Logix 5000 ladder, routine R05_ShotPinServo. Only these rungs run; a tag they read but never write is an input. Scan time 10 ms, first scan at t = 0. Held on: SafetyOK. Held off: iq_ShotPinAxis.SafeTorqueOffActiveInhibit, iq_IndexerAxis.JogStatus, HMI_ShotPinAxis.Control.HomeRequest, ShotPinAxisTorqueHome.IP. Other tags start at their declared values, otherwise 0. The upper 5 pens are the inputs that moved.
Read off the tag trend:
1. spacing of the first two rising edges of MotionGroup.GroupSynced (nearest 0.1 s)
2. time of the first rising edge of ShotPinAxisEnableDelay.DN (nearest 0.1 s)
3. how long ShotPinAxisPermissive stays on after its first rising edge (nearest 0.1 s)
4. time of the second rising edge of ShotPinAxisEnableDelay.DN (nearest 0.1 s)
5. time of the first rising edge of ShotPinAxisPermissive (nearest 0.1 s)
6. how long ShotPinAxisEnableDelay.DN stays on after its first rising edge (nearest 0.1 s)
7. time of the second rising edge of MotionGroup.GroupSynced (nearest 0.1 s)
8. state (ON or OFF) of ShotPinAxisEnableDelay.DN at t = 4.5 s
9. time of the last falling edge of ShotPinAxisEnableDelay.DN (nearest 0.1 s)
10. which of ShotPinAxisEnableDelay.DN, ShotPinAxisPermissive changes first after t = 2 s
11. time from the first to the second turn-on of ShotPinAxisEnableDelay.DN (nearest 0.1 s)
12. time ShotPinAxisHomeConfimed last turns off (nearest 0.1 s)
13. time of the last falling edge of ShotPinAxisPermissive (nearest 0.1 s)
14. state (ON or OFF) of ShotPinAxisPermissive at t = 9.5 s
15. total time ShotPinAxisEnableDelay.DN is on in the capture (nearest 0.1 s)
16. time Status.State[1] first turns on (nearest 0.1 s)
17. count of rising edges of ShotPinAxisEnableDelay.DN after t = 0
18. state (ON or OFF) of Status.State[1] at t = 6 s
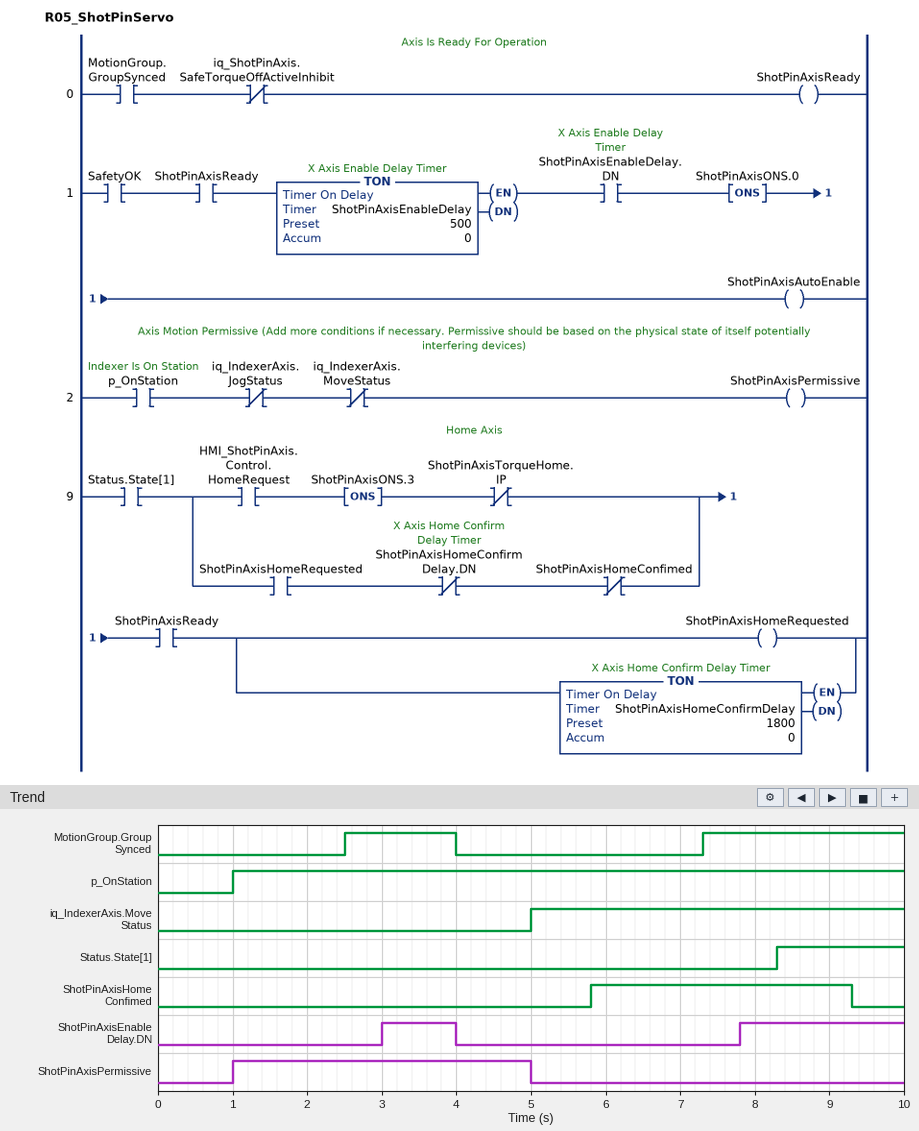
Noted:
4.8 s
3.0 s
4.0 s
7.8 s
1.0 s
1.0 s
7.3 s
OFF
4.0 s
ShotPinAxisEnableDelay.DN
4.8 s
9.3 s
5.0 s
OFF
3.2 s
8.3 s
2
OFF
